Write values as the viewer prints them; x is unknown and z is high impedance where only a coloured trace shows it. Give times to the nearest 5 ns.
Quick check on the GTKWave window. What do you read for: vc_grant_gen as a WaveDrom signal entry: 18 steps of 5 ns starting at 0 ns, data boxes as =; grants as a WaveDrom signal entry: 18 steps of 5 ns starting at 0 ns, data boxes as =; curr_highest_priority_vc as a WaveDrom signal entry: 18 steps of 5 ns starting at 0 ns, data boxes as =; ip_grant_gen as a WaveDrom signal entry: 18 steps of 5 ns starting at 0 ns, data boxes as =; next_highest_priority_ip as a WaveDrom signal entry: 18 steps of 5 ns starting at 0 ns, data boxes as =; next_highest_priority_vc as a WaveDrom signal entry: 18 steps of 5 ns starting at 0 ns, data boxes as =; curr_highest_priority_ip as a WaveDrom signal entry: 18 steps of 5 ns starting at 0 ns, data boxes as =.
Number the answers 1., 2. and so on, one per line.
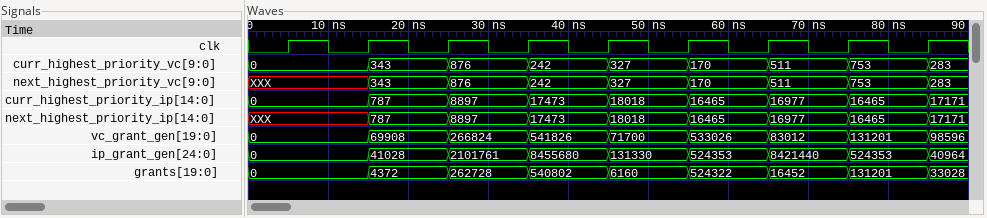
1. {name: 'vc_grant_gen', wave: '=..=.=.=.=.=.=.=.=', data: '0 69908 266824 541826 71700 533026 83012 131201 98596'}
2. {name: 'grants', wave: '=..=.=.=.=.=.=.=.=', data: '0 4372 262728 540802 6160 524322 16452 131201 33028'}
3. {name: 'curr_highest_priority_vc', wave: '=..=.=.=.=.=.=.=.=', data: '0 343 876 242 327 170 511 753 283'}
4. {name: 'ip_grant_gen', wave: '=..=.=.=.=.=.=.=.=', data: '0 41028 2101761 8455680 131330 524353 8421440 524353 40964'}
5. {name: 'next_highest_priority_ip', wave: 'x..=.=.=.=.=.=.=.=', data: '787 8897 17473 18018 16465 16977 16465 17171'}
6. {name: 'next_highest_priority_vc', wave: 'x..=.=.=.=.=.=.=.=', data: '343 876 242 327 170 511 753 283'}
7. {name: 'curr_highest_priority_ip', wave: '=..=.=.=.=.=.=.=.=', data: '0 787 8897 17473 18018 16465 16977 16465 17171'}
